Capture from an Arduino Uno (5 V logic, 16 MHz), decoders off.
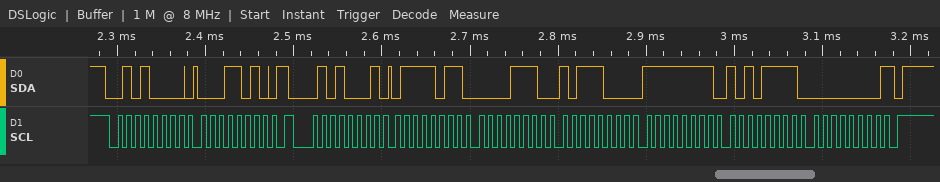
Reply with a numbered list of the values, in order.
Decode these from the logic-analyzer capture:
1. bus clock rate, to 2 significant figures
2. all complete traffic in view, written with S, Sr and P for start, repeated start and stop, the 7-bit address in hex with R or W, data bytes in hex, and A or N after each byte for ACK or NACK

1. 100 kHz
2. S 28W A 1A A Sr 28R A 7B A 0E A B8 A FF A AF A 00 N P
